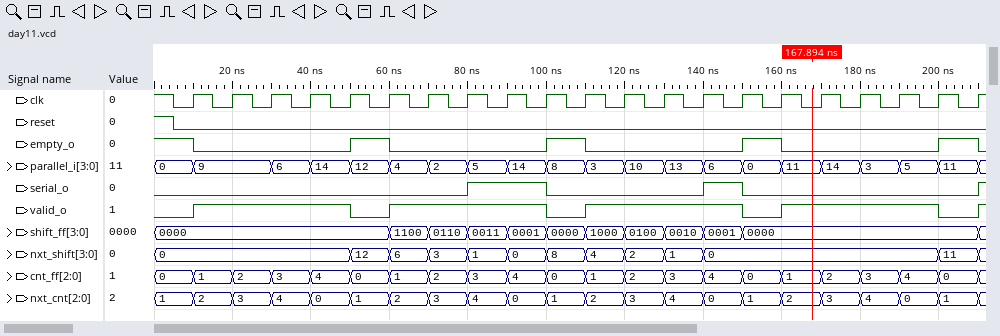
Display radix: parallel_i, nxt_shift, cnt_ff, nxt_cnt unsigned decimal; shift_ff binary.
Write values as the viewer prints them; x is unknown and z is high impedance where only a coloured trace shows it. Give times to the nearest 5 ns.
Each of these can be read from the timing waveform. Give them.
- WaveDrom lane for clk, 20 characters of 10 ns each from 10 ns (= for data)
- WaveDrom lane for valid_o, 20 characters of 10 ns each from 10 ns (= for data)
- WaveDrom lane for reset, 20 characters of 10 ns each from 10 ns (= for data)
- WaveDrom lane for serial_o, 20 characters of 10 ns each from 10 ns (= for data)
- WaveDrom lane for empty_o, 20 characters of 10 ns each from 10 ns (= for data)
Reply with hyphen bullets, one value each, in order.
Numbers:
- {name: 'clk', wave: 'p...................'}
- {name: 'valid_o', wave: '1...01...01...01...0'}
- {name: 'reset', wave: '0...................'}
- {name: 'serial_o', wave: '0......1.0...10.....'}
- {name: 'empty_o', wave: '0...10...10...10...1'}
